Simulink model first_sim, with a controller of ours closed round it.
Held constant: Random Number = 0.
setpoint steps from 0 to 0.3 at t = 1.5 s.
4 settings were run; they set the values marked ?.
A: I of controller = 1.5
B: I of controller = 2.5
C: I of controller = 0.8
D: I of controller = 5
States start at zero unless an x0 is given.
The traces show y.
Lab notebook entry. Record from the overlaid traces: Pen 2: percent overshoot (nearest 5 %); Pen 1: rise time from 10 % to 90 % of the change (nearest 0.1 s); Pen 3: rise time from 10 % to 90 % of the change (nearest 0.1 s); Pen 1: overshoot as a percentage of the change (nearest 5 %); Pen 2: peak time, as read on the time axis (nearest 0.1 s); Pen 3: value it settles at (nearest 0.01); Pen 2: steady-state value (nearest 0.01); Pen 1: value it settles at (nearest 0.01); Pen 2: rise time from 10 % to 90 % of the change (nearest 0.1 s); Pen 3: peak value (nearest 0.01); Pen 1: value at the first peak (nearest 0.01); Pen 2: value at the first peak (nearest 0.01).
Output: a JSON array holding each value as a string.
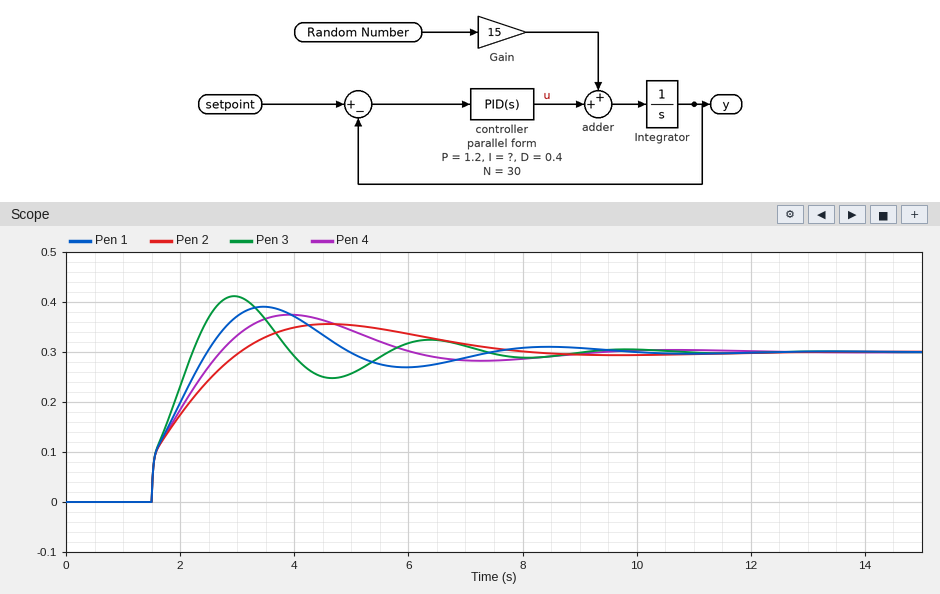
["20 %", "0.8 s", "0.6 s", "30 %", "4.6 s", "0.30", "0.30", "0.30", "1.2 s", "0.41", "0.39", "0.36"]
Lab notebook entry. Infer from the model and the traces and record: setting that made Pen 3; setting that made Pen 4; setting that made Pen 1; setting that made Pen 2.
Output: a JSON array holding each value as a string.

["D", "A", "B", "C"]
